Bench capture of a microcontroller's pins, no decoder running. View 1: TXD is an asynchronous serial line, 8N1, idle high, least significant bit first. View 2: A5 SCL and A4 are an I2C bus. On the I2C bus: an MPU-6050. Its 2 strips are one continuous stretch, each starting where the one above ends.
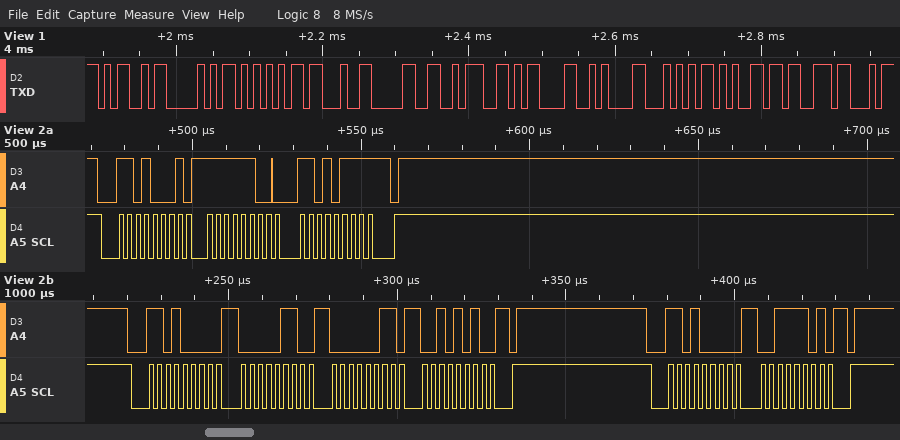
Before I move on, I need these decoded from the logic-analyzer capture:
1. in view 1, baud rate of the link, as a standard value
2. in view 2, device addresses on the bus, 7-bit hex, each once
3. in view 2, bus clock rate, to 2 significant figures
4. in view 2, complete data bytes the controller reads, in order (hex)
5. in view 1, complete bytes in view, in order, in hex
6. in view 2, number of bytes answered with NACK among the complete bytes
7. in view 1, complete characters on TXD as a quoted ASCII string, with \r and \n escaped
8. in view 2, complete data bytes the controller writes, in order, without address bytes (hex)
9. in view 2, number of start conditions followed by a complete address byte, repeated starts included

115200 baud
0x68
400 kHz
FC D7
4D 50 55 23 30 3A 0D 0A 54 65 73
1
"MPU#0:\r\nTes"
06 03 2A 3D
3
